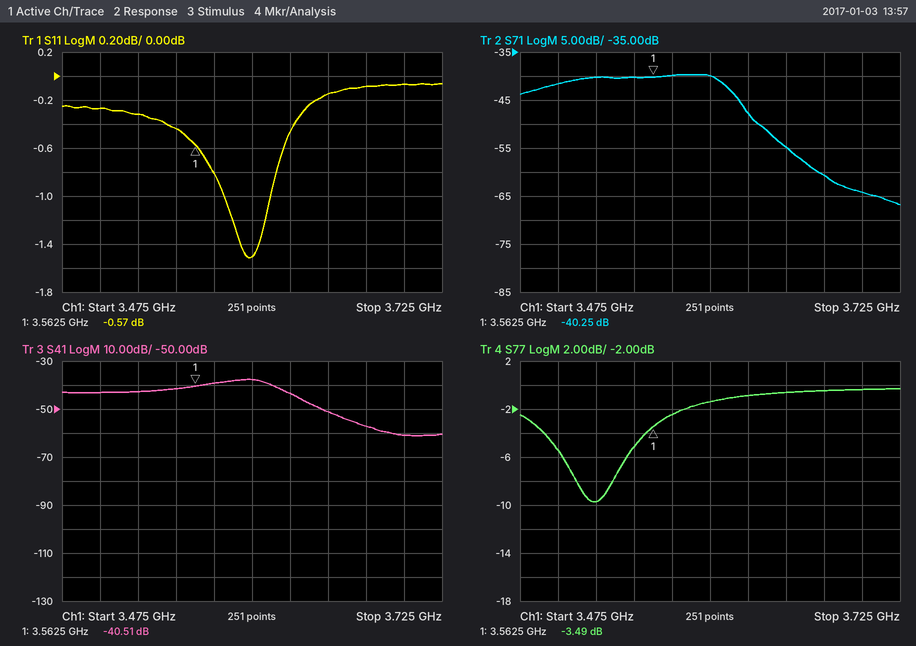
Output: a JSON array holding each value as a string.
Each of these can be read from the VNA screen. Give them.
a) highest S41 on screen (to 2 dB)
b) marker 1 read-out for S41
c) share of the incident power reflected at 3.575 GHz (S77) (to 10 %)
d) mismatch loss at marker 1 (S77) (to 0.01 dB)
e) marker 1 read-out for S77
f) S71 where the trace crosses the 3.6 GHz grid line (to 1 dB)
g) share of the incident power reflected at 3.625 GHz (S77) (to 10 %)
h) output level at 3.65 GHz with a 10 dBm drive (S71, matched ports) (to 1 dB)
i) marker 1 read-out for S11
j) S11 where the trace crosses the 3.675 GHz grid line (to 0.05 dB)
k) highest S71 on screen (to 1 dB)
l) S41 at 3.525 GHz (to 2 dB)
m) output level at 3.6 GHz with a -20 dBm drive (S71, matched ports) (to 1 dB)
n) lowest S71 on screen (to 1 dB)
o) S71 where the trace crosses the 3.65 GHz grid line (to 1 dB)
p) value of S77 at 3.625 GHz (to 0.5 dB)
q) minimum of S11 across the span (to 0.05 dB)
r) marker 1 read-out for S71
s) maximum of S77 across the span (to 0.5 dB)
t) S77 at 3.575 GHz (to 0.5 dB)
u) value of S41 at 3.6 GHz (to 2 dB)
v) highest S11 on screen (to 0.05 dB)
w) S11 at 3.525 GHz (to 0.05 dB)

["-38 dB", "-40.51 dB", "60 %", "2.58 dB", "-3.49 dB", "-40 dB", "80 %", "-45 dBm", "-0.57 dB", "-0.10 dB", "-40 dB", "-42 dB", "-60 dBm", "-67 dB", "-55 dB", "-1.0 dB", "-1.50 dB", "-40.25 dB", "-0.5 dB", "-2.5 dB", "-38 dB", "-0.05 dB", "-0.30 dB"]
